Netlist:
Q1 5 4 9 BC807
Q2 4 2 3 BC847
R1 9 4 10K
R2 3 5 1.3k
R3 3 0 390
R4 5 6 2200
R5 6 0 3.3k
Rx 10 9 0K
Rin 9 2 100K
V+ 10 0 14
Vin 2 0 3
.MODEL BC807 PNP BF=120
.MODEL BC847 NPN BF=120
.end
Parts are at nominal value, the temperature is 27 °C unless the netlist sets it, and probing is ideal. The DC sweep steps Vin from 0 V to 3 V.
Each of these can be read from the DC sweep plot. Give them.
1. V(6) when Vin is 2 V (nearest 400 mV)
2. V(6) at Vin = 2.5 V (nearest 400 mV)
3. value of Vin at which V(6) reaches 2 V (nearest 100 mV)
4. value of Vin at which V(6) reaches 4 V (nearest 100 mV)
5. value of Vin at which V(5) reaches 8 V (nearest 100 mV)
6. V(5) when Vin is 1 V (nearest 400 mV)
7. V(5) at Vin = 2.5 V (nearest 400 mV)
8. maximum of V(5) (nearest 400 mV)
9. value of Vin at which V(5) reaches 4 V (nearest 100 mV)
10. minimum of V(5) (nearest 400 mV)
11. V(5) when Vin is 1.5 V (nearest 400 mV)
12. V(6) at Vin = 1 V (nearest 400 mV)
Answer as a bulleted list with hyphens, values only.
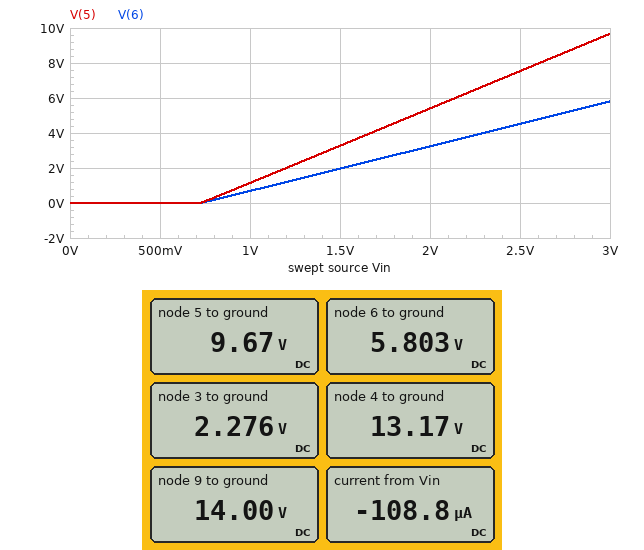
- 3.2 V
- 4.4 V
- 1.5 V
- 2.3 V
- 2.6 V
- 1.2 V
- 7.6 V
- 9.6 V
- 1.7 V
- 0 V
- 3.2 V
- 800 mV
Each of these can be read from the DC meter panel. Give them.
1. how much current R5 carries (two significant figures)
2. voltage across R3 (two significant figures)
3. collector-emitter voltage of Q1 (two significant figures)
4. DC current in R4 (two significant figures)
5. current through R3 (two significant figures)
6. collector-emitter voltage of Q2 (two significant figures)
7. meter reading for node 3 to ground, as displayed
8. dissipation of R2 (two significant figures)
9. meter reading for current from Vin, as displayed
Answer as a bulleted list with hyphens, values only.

- 1.8 mA
- 2.3 V
- -4.3 V
- 1.8 mA
- 5.8 mA
- 11 V
- 2.276 V
- 42 mW
- -108.8 µA
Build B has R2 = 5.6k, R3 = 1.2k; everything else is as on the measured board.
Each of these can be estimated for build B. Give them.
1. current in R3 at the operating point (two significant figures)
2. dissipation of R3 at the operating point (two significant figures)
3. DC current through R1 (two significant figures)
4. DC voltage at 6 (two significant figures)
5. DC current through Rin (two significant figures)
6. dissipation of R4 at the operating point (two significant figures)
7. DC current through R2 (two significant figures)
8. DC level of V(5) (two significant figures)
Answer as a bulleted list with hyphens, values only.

- 1.9 mA
- 4.3 mW
- 81 µA
- 7.4 V
- 110 µA
- 11 mW
- 1.8 mA
- 12 V
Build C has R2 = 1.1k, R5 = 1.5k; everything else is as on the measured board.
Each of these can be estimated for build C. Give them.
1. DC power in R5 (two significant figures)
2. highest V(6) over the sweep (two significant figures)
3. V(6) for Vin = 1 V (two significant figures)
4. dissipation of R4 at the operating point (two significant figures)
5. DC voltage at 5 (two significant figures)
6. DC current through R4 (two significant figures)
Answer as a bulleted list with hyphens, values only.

- 8.0 mW
- 3.5 V
- 410 mV
- 12 mW
- 8.5 V
- 2.3 mA
